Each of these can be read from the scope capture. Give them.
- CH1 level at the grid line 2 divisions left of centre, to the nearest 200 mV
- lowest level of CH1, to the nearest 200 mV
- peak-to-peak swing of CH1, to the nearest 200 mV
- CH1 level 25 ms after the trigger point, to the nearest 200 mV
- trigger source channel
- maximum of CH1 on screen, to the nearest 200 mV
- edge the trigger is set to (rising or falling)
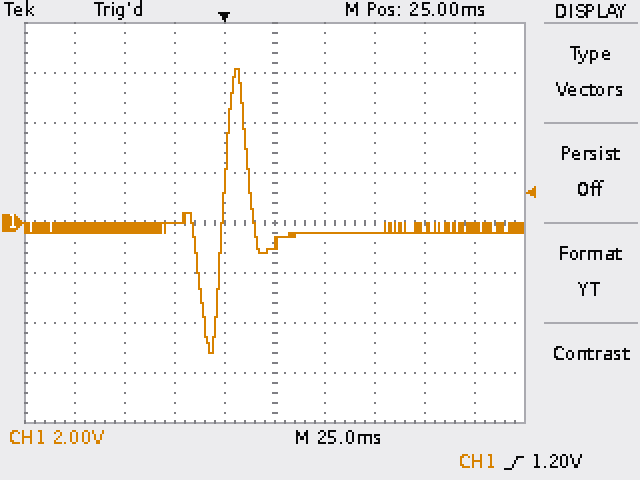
0.0 V
-5.2 V
11.4 V
-800 mV
CH1
6.2 V
rising
